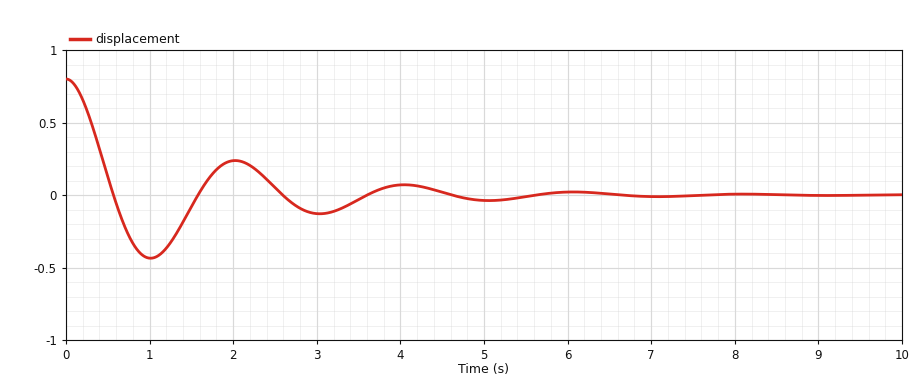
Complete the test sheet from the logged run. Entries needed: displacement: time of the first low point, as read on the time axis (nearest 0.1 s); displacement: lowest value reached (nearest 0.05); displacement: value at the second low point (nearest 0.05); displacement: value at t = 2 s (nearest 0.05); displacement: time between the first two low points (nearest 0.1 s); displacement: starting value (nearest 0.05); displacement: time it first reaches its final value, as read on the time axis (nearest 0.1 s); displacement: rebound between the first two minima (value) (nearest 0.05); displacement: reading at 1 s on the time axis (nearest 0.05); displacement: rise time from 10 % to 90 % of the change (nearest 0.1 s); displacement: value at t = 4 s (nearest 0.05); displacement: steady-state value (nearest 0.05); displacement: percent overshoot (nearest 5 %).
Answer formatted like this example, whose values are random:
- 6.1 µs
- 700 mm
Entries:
- 1.0 s
- -0.45
- -0.15
- 0.25
- 2.0 s
- 0.80
- 0.6 s
- 0.25
- -0.45
- 0.4 s
- 0.05
- 0.00
- 55 %
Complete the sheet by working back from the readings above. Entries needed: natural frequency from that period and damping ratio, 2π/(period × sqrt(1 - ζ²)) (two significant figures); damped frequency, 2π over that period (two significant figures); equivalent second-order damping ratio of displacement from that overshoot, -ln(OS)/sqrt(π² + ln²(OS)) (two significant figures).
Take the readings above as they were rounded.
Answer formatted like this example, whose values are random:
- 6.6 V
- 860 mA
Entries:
- 3.2 rad/s
- 3.1 rad/s
- 0.19
